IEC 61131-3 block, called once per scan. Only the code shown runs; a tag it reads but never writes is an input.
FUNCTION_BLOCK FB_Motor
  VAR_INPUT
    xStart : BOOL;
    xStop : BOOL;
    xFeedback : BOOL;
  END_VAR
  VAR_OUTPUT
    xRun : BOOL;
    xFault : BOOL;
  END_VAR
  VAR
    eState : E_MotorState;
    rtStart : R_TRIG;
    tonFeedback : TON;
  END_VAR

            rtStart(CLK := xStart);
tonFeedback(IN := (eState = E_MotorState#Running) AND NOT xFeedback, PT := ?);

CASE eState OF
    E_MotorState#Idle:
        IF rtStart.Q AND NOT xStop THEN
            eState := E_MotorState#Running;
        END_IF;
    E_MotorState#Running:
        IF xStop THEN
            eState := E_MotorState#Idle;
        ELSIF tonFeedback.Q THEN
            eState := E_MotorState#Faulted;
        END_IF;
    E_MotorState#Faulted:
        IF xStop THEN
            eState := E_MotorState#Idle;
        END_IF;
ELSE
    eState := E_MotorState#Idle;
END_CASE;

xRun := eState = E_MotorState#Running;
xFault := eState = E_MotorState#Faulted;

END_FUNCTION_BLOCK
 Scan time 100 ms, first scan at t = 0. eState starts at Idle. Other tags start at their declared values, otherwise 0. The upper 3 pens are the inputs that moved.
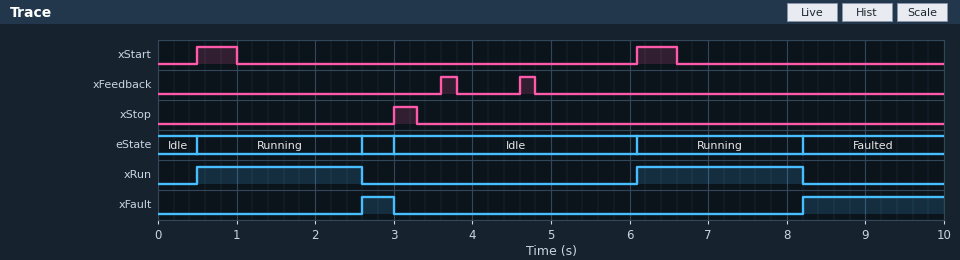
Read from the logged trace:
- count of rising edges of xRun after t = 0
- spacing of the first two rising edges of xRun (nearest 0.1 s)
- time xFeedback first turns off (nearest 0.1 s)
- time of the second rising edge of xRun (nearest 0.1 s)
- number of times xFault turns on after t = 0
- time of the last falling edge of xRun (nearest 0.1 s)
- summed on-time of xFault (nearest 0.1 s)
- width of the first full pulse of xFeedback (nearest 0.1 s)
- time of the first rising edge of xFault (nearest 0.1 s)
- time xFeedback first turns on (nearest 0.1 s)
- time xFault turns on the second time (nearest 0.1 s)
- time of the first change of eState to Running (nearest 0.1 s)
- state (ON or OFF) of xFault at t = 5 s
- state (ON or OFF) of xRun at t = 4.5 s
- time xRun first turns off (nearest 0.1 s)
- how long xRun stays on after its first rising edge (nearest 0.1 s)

2
5.6 s
3.8 s
6.1 s
2
8.2 s
2.2 s
0.2 s
2.6 s
3.6 s
8.2 s
0.5 s
OFF
OFF
2.6 s
2.1 s
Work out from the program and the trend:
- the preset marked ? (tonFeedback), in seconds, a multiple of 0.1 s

2.0 s
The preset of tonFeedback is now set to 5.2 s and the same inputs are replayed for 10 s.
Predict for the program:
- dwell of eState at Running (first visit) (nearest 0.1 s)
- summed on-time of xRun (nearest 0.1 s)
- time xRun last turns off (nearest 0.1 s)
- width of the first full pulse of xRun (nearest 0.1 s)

2.5 s
6.4 s
3.0 s
2.5 s
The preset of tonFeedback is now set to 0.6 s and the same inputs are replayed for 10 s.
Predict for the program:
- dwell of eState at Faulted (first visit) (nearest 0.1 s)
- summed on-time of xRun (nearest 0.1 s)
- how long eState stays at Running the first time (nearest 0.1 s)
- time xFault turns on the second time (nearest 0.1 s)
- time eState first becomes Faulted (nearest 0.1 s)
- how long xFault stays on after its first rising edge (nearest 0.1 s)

1.8 s
1.4 s
0.7 s
6.8 s
1.2 s
1.8 s
